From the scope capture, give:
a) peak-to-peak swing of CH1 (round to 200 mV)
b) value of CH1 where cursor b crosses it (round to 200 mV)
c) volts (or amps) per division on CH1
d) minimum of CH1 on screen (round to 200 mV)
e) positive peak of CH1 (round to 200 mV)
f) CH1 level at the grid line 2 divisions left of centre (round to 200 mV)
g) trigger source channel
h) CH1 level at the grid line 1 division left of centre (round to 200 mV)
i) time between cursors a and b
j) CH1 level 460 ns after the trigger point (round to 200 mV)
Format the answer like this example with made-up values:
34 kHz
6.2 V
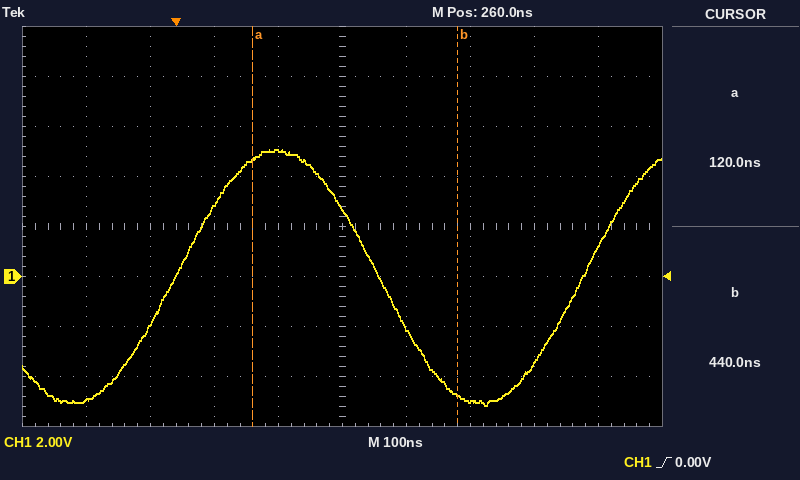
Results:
10.2 V
-4.8 V
2 V
-5.2 V
5.0 V
2.8 V
CH1
5.0 V
320 ns
-5.0 V
